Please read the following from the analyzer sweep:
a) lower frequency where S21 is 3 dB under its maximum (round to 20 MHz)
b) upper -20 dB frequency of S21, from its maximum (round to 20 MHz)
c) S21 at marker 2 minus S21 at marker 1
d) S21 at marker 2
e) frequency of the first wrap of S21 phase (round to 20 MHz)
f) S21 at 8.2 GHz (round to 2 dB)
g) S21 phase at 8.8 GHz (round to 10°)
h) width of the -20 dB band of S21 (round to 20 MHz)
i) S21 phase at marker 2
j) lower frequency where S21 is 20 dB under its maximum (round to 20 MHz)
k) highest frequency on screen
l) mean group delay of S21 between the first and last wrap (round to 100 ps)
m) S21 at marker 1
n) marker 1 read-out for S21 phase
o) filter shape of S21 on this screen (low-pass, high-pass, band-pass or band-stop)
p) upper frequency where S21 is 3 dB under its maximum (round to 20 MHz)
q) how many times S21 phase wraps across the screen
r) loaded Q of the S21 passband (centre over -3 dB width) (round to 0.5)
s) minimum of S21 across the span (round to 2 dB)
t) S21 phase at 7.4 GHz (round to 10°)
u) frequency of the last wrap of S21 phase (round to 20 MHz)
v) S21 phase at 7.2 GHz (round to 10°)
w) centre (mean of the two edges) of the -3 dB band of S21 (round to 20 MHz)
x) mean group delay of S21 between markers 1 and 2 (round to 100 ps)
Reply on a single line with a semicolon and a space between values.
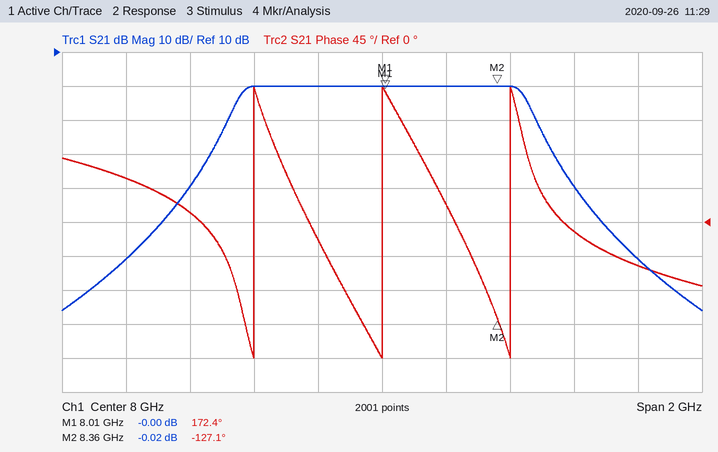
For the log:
7.56 GHz; 8.54 GHz; -0.02 dB; -0.02 dB; 7.60 GHz; 0 dB; -60°; 1.08 GHz; -127.1°; 7.46 GHz; 9 GHz; 2.5 ns; -0.00 dB; 172.4°; band-pass; 8.44 GHz; 3; 9.0; -66 dB; 10°; 8.40 GHz; 60°; 8.00 GHz; 2.4 ns
